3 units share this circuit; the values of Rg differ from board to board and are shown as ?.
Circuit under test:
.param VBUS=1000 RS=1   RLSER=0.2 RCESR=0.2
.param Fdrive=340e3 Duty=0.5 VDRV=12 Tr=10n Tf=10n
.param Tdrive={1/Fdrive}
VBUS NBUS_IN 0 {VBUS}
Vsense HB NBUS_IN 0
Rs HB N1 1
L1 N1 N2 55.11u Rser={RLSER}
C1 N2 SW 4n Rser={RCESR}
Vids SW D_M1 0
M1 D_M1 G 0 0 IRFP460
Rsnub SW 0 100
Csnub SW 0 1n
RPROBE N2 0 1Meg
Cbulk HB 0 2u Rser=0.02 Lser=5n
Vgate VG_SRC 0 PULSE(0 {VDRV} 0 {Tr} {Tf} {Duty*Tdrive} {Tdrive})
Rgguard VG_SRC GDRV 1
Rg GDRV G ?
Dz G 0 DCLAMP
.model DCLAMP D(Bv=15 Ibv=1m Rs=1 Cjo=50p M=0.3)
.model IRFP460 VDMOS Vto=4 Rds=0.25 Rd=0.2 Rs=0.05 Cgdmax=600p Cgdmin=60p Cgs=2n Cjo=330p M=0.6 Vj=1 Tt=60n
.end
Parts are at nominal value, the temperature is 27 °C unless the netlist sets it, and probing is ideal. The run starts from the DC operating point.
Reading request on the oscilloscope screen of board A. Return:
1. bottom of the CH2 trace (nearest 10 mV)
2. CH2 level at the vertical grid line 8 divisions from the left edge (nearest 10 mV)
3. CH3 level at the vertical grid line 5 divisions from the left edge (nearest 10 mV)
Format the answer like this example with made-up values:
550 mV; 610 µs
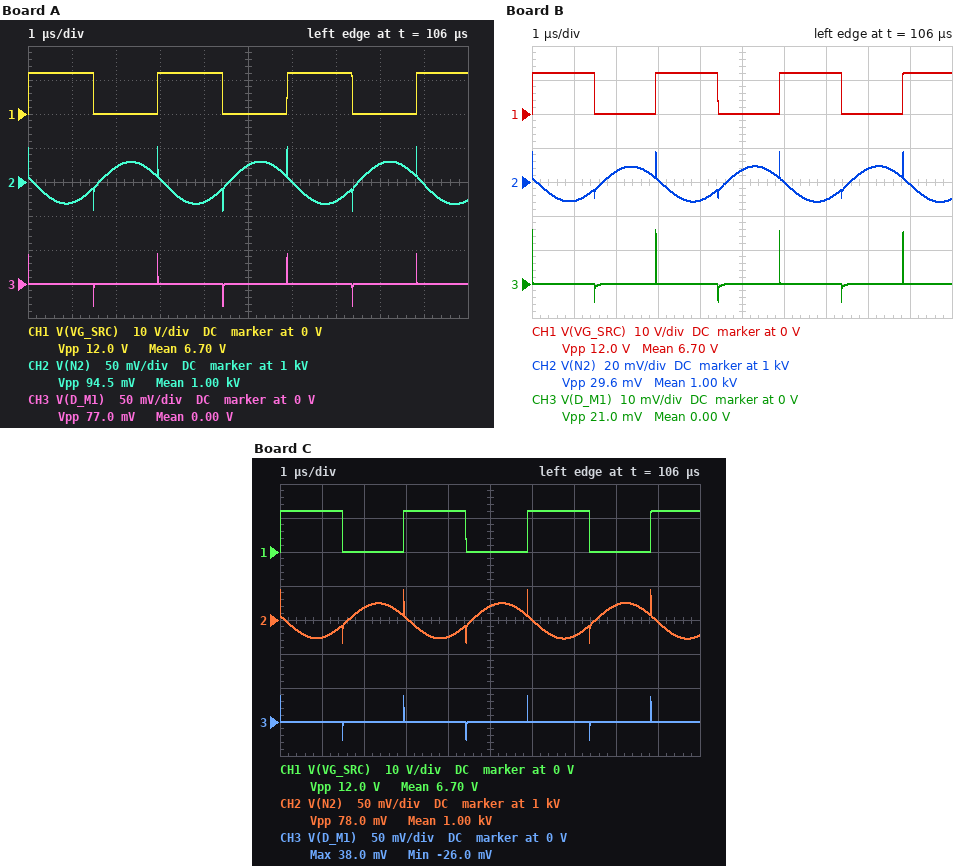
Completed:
999.96 V; 1.00003 kV; 0 V
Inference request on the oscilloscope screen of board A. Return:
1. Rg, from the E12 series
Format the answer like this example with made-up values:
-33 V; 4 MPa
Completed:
3.3 Ω
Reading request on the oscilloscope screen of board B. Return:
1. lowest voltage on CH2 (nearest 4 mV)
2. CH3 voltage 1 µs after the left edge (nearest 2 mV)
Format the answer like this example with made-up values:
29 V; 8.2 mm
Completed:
999.988 V; 0 V
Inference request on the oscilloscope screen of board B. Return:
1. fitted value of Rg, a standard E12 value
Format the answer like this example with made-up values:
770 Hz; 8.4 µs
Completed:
33 Ω
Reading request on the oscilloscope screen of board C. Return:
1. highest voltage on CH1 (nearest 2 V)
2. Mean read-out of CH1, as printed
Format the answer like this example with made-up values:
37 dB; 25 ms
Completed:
12 V; 6.70 V
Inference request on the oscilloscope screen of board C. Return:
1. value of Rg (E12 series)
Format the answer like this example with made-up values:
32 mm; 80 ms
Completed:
4.7 Ω
